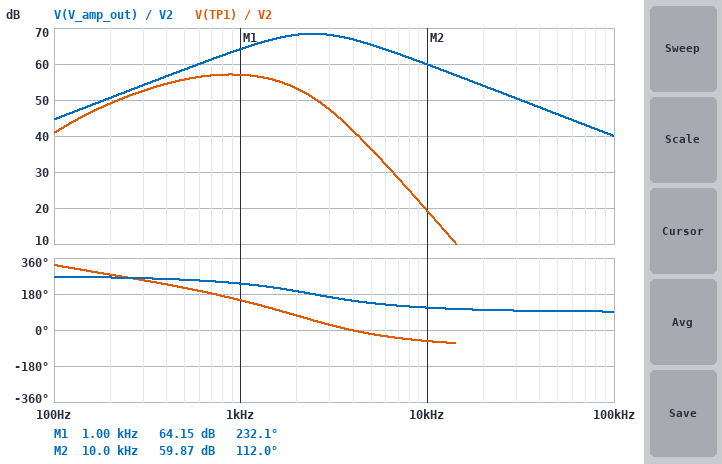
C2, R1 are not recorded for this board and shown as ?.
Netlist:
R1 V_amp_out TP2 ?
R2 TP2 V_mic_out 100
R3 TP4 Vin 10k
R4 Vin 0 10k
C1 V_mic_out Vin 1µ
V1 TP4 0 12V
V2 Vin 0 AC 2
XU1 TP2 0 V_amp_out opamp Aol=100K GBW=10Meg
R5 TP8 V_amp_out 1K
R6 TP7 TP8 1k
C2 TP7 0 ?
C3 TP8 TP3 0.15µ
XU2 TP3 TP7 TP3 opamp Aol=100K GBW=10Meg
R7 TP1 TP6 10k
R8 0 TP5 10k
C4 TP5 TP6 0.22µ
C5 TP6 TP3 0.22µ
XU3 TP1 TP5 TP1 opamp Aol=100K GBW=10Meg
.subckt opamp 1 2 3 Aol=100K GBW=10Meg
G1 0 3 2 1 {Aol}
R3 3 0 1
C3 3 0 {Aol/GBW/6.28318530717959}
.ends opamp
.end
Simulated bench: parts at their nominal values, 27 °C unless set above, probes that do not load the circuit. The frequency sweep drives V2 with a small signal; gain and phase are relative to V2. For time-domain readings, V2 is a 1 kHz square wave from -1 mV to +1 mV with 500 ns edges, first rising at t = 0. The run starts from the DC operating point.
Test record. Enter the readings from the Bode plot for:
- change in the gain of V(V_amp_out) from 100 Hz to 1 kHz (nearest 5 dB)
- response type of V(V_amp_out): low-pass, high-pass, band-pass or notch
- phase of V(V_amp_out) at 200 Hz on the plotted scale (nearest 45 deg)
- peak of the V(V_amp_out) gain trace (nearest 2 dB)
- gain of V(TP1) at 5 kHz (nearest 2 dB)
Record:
20 dB
band-pass
270 deg
68 dB
36 dB
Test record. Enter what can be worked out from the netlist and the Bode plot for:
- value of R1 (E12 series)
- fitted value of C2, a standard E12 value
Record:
270 kΩ
180 nF
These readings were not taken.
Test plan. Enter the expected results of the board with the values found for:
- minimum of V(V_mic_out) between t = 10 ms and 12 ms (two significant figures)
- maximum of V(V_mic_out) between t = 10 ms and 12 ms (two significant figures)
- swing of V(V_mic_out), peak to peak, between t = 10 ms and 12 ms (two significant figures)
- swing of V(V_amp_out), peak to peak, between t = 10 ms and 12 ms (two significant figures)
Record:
-2.0 mV
2.0 mV
4.0 mV
7.1 V
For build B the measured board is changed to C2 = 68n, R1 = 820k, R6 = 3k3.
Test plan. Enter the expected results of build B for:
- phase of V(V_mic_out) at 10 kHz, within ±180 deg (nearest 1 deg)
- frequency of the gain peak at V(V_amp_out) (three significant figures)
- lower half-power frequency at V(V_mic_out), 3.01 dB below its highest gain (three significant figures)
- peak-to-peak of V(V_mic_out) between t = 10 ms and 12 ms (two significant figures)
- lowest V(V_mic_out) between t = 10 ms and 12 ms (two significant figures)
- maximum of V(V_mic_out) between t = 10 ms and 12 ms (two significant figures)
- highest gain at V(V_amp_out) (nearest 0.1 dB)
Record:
0 deg
1.39 kHz
1.03 kHz
4.6 mV
-2.3 mV
2.3 mV
77.6 dB
